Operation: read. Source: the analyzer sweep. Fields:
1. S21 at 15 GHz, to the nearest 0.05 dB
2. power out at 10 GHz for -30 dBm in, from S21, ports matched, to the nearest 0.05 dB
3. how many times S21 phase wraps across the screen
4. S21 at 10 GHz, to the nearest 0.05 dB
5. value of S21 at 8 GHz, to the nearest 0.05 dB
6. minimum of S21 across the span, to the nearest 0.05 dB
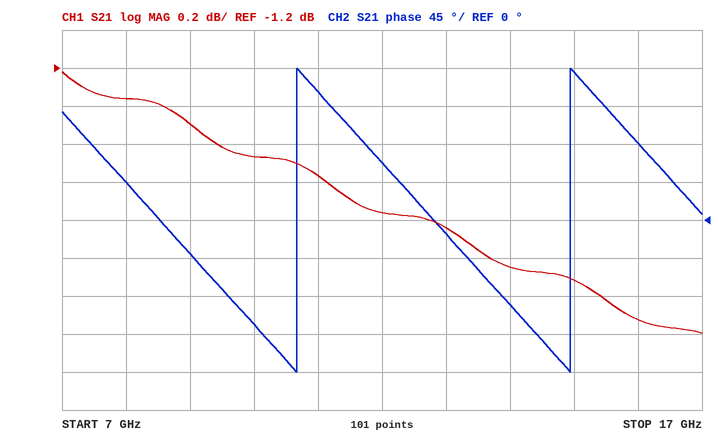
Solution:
-2.30 dB
-31.65 dBm
2
-1.65 dB
-1.35 dB
-2.60 dB
